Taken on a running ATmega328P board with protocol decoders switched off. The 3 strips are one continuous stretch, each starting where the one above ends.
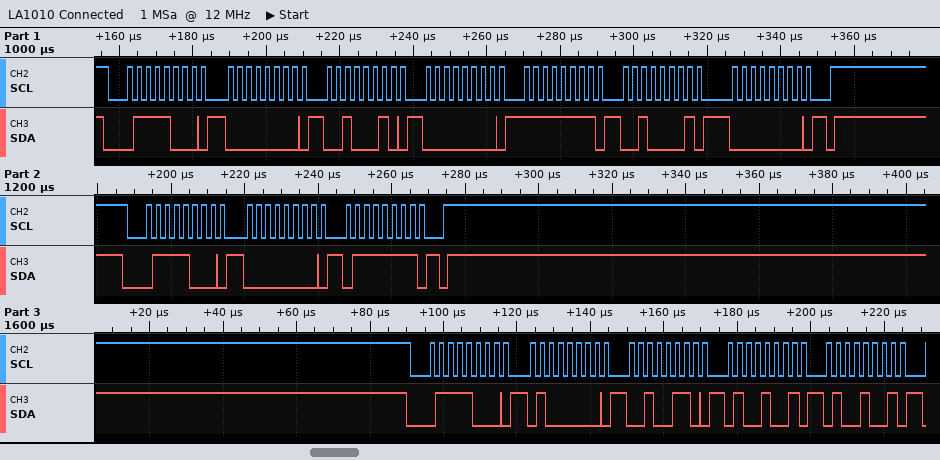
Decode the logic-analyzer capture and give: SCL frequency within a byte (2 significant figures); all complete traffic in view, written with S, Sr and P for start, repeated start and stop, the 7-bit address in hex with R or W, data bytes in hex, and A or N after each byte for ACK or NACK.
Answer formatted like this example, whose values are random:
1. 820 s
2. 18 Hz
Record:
1. 400 kHz
2. S 3CW A 00 A 22 A 00 A FF A 21 A 00 A P S 3CW A 00 A 7F A P S 3CW A 40 A 26 A 49 A 49 A
